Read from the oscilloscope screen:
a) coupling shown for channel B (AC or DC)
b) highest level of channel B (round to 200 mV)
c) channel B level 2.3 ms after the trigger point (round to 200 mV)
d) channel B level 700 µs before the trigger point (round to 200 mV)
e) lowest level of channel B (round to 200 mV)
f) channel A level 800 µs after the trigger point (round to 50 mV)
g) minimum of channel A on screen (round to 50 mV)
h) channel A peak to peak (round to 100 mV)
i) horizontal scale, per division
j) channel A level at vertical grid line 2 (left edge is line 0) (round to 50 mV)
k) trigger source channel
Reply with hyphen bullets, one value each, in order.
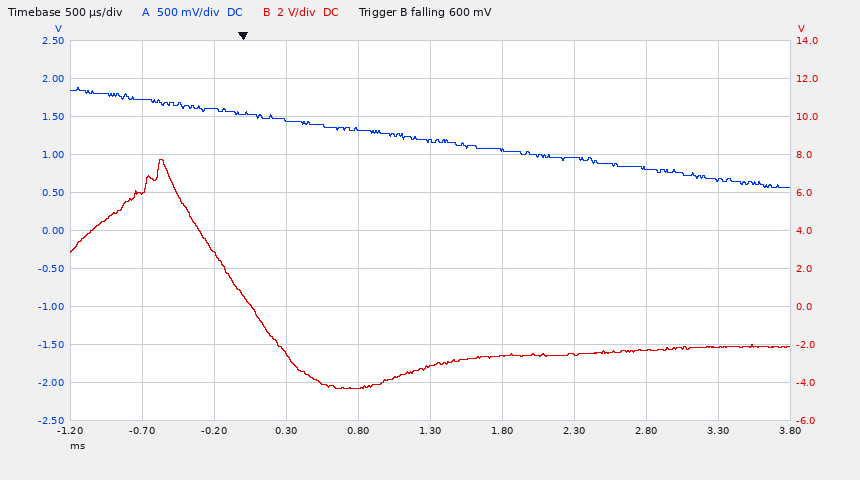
- DC
- 7.8 V
- -2.6 V
- 6.0 V
- -4.4 V
- 1.35 V
- 550 mV
- 1.30 V
- 500 µs
- 1.60 V
- channel B
